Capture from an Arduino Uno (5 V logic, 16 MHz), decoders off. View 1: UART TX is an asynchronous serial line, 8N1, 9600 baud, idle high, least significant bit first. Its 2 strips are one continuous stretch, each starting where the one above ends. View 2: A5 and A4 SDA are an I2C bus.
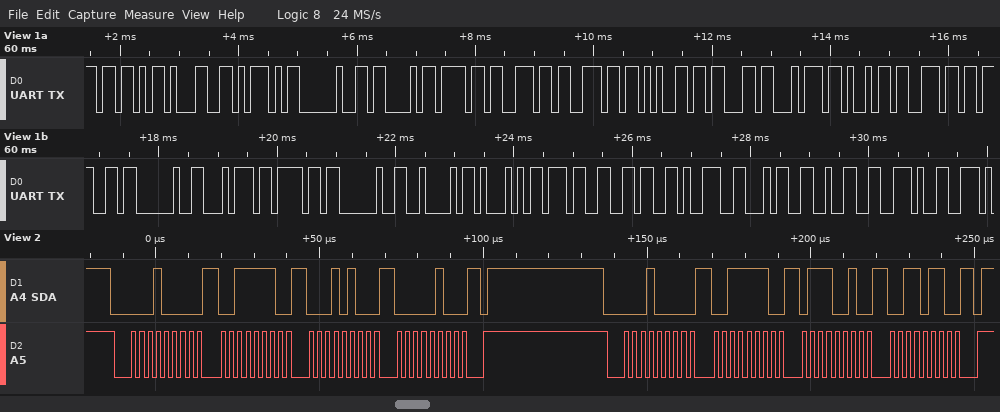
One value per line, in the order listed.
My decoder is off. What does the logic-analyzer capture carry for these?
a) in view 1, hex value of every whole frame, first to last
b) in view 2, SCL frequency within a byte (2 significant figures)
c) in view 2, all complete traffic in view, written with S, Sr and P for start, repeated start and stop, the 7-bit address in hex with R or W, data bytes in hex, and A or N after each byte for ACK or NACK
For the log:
0x5B 0x31 0x5D 0x20 0x43 0x6F 0x6E 0x6E 0x65 0x63 0x74 0x69 0x6E 0x67 0x20 0x74 0x6F 0x20 0x42 0x51 0x37 0x36 0x39 0x34 0x32 0x2E
400 kHz
S 08W A 3E A 14 A 04 A P S 08W A 3E A 72 A 36 A P
